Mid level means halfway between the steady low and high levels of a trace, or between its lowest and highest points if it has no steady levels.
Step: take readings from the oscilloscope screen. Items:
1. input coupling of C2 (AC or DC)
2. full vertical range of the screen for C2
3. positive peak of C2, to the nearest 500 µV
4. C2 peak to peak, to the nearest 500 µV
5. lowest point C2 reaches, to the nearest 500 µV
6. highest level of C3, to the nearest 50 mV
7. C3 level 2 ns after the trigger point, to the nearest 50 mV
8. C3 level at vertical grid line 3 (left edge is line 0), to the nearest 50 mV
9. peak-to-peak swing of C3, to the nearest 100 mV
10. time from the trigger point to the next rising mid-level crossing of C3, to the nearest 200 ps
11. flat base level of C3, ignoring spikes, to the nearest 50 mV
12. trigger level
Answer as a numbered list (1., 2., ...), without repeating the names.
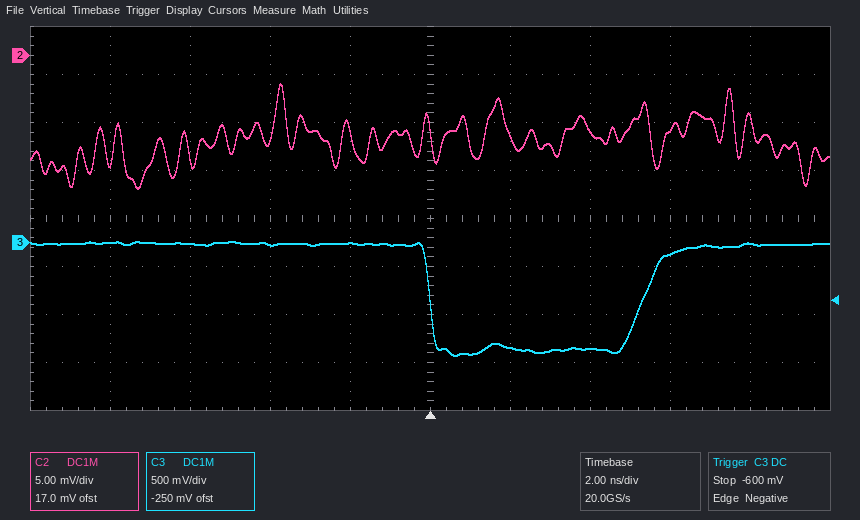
1. DC
2. 40 mV
3. -3.0 mV
4. 11.0 mV
5. -14.0 mV
6. 0 mV
7. -1.10 V
8. 0 mV
9. 1.20 V
10. 5.4 ns
11. -1.10 V
12. -600 mV
